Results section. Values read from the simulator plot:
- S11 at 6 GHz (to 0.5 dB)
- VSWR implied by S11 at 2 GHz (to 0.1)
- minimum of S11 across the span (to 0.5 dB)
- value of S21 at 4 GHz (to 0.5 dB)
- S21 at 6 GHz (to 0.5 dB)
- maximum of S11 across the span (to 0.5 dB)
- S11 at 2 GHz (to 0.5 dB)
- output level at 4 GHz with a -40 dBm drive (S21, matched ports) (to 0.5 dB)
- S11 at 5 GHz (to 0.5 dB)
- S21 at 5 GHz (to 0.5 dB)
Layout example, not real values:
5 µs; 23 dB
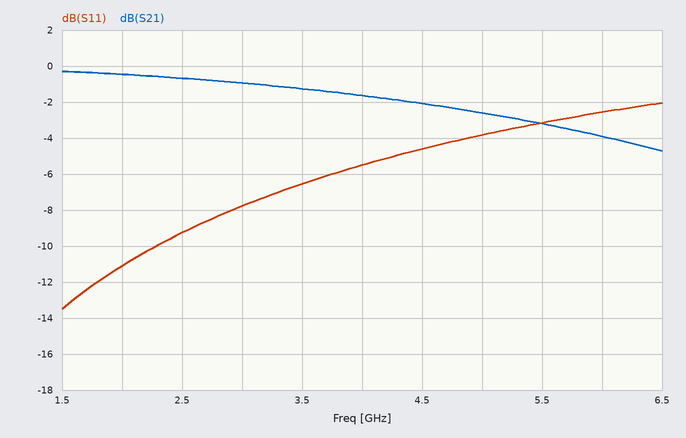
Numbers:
-2.5 dB; 1.8; -13.5 dB; -1.5 dB; -4.0 dB; -2.0 dB; -11.0 dB; -41.5 dBm; -4.0 dB; -2.5 dB
